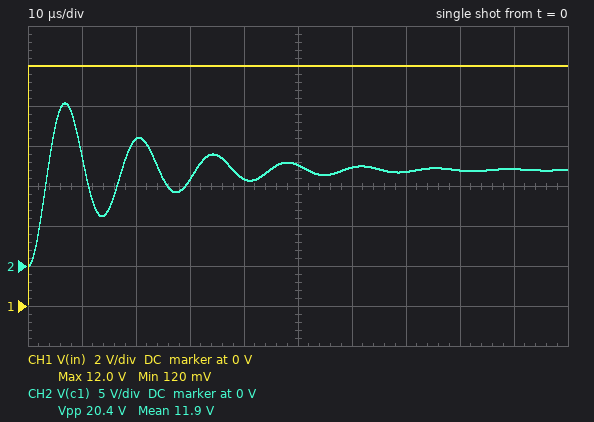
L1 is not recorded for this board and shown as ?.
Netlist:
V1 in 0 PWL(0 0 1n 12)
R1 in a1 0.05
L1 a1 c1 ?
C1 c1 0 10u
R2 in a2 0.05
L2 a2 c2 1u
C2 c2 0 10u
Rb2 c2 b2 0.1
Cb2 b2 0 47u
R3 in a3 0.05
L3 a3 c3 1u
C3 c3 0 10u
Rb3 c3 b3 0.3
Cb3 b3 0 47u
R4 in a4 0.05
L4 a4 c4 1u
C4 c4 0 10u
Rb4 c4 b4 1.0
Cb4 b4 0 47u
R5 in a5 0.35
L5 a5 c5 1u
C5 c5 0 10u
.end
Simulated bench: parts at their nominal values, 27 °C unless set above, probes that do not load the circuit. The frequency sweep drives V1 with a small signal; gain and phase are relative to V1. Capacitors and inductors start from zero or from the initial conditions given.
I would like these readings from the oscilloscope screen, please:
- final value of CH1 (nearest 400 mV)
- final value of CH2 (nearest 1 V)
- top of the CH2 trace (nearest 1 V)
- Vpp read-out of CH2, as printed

12.0 V
12 V
20 V
20.4 V
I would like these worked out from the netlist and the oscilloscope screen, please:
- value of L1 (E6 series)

470 nH
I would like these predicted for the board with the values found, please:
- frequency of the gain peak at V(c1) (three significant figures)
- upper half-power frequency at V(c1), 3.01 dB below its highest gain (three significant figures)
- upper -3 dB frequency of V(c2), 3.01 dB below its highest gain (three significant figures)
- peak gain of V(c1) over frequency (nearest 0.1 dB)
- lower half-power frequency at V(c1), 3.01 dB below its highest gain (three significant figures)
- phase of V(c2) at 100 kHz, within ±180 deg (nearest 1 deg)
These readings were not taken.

72.4 kHz
80.5 kHz
27.6 kHz
12.8 dB
63.3 kHz
-126 deg
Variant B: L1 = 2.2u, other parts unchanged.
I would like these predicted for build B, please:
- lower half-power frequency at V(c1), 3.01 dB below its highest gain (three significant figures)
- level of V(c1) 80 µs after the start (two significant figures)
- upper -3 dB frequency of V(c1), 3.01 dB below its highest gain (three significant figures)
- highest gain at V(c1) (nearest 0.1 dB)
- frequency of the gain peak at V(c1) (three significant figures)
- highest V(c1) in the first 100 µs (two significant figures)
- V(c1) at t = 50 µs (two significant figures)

32.0 kHz
13 V
35.6 kHz
19.5 dB
33.8 kHz
22 V
15 V
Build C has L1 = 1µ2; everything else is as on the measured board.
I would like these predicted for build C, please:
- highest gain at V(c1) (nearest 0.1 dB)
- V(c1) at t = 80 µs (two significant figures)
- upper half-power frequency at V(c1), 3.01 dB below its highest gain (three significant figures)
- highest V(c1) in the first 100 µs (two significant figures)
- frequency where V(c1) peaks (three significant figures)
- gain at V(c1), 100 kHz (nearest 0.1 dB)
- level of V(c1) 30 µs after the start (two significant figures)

16.8 dB
13 V
48.9 kHz
22 V
45.7 kHz
-11.5 dB
16 V
